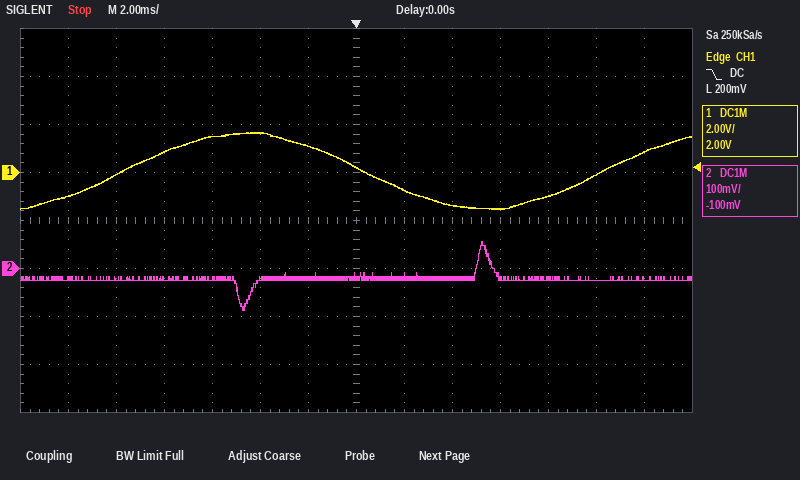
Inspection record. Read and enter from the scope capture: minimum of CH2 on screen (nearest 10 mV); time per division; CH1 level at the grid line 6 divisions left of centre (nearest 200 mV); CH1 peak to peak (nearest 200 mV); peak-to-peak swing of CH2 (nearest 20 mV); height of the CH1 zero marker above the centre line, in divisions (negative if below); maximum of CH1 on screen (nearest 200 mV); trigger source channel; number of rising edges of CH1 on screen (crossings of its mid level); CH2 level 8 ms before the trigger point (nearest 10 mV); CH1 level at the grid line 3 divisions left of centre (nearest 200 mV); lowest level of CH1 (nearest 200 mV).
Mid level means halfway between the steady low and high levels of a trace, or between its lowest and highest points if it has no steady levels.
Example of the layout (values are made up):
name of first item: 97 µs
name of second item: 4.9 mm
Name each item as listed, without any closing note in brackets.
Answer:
minimum of CH2 on screen: -90 mV
time per division: 2 ms
CH1 level at the grid line 6 divisions left of centre: -1.0 V
CH1 peak to peak: 3.2 V
peak-to-peak swing of CH2: 140 mV
height of the CH1 zero marker above the centre line, in divisions: +1.0 div
maximum of CH1 on screen: 1.6 V
trigger source channel: CH1
number of rising edges of CH1 on screen: 2
CH2 level 8 ms before the trigger point: -20 mV
CH1 level at the grid line 3 divisions left of centre: 1.4 V
lowest level of CH1: -1.6 V
